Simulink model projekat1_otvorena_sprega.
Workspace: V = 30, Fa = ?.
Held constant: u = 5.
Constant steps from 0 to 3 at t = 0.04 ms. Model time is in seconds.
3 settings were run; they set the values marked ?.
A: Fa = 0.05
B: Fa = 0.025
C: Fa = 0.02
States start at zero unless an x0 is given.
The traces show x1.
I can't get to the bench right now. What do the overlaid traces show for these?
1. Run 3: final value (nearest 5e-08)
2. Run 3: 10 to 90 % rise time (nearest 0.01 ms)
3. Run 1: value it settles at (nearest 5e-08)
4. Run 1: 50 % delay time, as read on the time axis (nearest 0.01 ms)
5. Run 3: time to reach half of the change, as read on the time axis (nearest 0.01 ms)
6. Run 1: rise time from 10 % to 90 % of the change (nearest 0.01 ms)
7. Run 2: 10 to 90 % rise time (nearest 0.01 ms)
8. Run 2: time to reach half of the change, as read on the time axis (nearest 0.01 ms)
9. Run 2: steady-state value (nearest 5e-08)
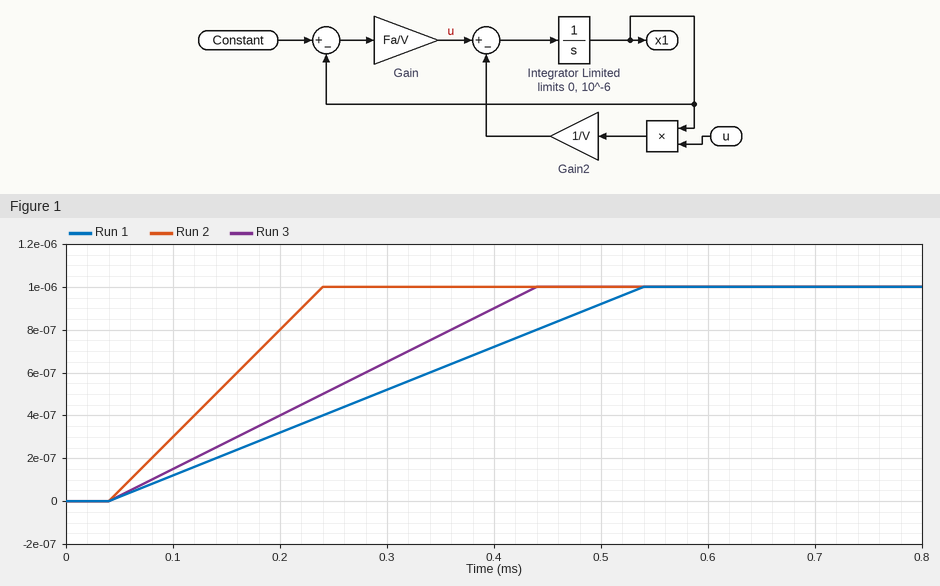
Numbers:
0.00000100
0.32 ms
0.00000100
0.29 ms
0.24 ms
0.40 ms
0.16 ms
0.14 ms
0.00000100
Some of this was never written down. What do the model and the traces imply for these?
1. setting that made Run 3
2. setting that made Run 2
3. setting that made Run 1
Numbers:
B
A
C
